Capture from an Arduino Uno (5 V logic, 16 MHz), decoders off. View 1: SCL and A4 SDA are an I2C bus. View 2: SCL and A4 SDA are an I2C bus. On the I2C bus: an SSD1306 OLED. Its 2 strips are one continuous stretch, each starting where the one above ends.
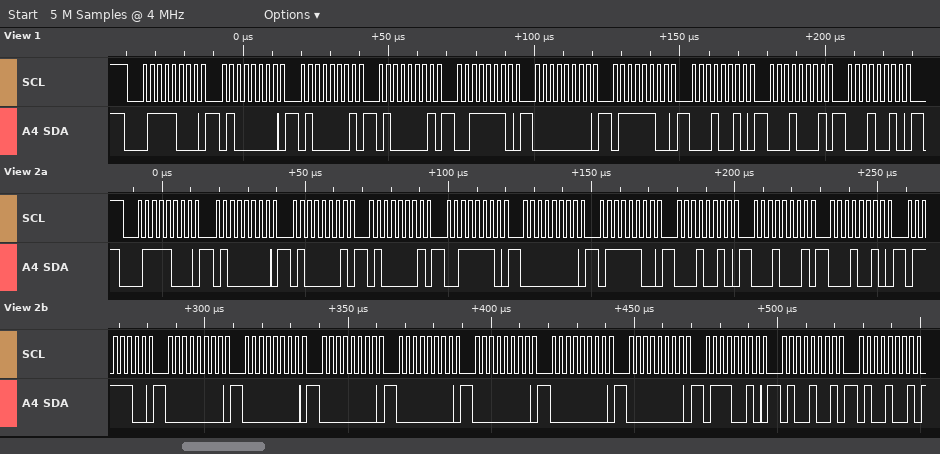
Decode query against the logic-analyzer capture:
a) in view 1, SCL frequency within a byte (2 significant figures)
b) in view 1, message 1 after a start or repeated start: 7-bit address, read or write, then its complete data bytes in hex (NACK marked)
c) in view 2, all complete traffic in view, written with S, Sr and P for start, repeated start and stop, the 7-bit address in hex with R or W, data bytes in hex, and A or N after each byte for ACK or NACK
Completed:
400 kHz
0x3C write: 40 41 41 3E 00 7C 12 11 12
S 3CW A 40 A 41 A 41 A 3E A 00 A 7C A 12 A 11 A 12 A 7C A 00 A 00 A 00 A 00 A 00 A 00 A 00 A 72 A 49 A 49 A
